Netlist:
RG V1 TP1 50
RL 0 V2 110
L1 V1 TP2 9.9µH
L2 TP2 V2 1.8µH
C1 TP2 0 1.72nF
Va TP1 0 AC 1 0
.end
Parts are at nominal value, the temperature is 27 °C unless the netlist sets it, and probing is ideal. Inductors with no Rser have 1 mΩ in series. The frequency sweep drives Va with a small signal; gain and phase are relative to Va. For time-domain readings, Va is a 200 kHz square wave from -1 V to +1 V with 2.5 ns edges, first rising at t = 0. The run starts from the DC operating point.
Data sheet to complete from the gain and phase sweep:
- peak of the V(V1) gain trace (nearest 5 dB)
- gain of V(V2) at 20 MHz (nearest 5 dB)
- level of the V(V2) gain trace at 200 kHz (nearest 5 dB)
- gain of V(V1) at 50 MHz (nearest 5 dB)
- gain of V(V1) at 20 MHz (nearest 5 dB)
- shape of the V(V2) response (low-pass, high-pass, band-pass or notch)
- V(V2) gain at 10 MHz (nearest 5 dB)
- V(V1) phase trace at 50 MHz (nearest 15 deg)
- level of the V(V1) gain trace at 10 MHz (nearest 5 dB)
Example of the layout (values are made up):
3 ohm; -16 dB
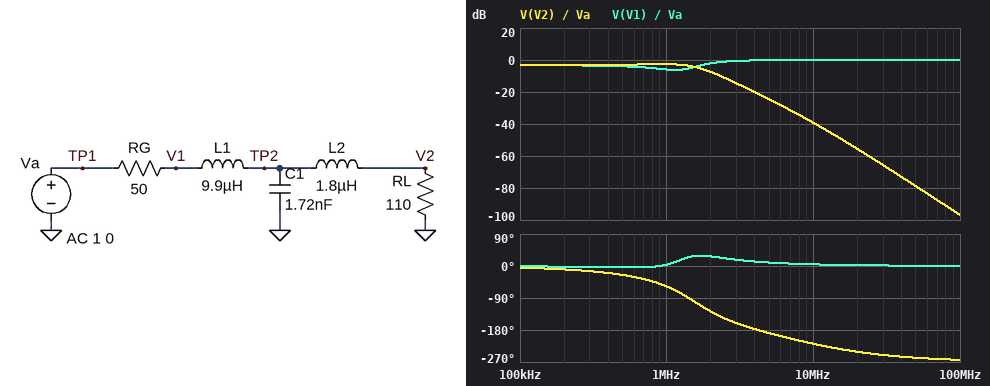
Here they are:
0 dB; -55 dB; -5 dB; 0 dB; 0 dB; low-pass; -40 dB; 0 deg; 0 dB
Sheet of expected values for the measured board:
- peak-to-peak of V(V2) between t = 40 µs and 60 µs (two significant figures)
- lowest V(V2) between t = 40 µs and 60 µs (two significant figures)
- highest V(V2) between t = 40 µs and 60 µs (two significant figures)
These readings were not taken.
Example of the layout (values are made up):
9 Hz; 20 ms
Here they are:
1.7 V; -860 mV; 860 mV
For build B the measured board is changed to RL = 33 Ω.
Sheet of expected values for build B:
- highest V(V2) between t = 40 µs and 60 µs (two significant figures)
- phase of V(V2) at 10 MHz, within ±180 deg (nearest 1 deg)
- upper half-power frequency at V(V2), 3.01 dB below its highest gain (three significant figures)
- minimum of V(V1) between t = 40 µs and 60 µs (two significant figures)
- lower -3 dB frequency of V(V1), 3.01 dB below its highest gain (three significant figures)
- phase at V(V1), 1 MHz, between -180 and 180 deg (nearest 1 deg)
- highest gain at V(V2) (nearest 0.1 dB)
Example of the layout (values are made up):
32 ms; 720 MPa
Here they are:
400 mV; 112 deg; 1.68 MHz; -1.6 V; 1.17 MHz; 24 deg; -8.0 dB
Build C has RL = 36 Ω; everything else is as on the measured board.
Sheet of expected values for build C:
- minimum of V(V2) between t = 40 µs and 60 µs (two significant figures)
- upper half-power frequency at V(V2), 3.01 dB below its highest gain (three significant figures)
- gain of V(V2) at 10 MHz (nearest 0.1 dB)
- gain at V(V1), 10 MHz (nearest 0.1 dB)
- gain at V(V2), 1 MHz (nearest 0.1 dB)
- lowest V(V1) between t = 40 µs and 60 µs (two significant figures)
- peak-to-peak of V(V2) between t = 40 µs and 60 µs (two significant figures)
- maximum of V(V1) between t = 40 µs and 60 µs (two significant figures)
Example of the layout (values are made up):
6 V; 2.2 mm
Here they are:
-420 mV; 1.73 MHz; -46.1 dB; 0 dB; -9.0 dB; -1.6 V; 840 mV; 1.6 V
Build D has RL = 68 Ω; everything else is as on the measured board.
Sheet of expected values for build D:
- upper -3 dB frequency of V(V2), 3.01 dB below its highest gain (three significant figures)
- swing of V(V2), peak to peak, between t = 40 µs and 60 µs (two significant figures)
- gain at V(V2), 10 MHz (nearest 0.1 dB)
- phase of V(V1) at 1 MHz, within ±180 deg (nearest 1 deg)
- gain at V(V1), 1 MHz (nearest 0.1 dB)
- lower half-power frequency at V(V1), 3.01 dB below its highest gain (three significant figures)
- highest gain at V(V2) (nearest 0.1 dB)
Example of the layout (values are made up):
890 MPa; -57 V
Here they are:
1.85 MHz; 1.3 V; -41.7 dB; 14 deg; -4.9 dB; 1.70 MHz; -4.8 dB
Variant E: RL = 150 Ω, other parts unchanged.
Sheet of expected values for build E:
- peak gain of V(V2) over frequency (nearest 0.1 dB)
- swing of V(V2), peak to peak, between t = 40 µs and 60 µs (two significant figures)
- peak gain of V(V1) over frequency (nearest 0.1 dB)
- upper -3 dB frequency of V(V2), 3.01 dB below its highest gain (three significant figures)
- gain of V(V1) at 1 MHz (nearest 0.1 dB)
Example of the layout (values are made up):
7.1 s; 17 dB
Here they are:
-1.3 dB; 2.0 V; 0 dB; 1.68 MHz; -6.5 dB
